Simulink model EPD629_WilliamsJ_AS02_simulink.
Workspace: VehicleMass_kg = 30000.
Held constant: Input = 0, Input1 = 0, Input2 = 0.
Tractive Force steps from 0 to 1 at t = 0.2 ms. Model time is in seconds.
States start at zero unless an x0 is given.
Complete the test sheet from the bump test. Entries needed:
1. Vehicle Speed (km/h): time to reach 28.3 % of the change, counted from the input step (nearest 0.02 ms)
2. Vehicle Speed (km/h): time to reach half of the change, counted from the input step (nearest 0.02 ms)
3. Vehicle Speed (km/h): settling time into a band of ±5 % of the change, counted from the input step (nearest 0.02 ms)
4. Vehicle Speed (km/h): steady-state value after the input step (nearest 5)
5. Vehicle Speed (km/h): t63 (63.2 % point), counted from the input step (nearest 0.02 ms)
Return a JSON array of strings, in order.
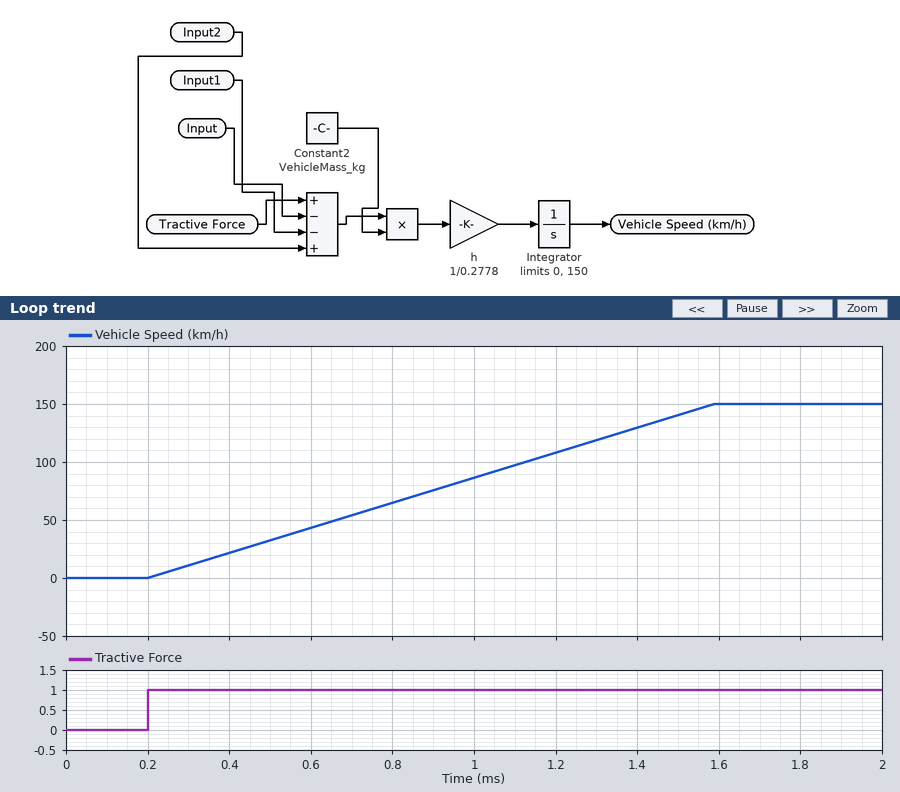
["0.40 ms", "0.70 ms", "1.32 ms", "150", "0.88 ms"]
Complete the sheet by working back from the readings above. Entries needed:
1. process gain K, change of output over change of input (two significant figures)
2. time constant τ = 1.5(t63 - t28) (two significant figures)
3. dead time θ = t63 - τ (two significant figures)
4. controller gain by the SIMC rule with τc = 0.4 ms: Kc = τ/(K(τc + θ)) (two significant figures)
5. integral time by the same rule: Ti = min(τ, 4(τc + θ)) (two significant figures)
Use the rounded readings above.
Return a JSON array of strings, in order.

["150", "0.72 ms", "0.16 ms", "0.0086", "0.72 ms"]
